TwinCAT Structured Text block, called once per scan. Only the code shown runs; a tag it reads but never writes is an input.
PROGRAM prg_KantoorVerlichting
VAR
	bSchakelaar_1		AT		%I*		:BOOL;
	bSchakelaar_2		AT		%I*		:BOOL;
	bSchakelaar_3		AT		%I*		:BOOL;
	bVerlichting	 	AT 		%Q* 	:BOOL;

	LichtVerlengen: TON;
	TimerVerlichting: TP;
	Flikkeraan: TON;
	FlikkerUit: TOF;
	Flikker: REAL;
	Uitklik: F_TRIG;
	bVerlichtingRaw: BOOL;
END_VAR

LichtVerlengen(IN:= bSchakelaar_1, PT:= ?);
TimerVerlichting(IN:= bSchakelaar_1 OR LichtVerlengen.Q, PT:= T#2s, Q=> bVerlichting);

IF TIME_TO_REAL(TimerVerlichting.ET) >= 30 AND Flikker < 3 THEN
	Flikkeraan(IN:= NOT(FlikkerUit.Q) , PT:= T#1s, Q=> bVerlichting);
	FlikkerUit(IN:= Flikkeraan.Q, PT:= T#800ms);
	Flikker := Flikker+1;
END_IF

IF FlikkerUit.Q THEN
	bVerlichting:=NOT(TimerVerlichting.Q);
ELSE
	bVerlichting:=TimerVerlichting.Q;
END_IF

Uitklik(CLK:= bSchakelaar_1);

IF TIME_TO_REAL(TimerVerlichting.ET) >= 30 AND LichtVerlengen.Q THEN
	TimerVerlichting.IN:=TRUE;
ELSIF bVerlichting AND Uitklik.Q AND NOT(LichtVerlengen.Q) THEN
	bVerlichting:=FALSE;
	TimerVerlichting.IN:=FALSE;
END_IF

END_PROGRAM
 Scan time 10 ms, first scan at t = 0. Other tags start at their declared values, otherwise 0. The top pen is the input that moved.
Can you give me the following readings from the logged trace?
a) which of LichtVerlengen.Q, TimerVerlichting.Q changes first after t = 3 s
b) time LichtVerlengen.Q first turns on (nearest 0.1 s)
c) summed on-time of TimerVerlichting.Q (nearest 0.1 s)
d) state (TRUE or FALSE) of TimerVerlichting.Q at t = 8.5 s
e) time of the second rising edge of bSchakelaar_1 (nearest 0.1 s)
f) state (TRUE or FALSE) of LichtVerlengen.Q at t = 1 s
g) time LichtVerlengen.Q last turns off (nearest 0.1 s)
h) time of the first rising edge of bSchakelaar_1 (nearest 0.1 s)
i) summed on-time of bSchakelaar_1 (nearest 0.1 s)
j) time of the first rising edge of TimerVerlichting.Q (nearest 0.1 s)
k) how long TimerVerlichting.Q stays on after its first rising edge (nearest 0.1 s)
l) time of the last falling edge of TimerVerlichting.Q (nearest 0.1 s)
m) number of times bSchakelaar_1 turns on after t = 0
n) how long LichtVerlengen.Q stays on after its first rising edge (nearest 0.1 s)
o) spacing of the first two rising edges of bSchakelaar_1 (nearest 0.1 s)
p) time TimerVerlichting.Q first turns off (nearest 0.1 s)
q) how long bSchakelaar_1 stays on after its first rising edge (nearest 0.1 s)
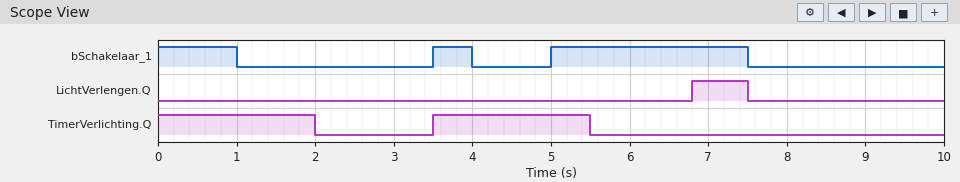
TimerVerlichting.Q
6.8 s
4.0 s
FALSE
5.0 s
FALSE
7.5 s
3.5 s
4.0 s
3.5 s
2.0 s
5.5 s
2
0.7 s
1.5 s
2.0 s
0.5 s
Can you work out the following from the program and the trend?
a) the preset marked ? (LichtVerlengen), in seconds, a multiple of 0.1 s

1.8 s
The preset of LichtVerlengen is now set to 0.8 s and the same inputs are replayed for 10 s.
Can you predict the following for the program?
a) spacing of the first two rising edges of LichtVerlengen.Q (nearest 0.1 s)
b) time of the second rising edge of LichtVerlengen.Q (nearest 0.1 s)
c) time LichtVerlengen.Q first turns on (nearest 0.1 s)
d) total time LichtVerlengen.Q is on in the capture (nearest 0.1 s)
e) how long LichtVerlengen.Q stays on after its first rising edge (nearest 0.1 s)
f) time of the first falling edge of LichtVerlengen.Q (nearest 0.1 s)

5.0 s
5.8 s
0.8 s
1.9 s
0.2 s
1.0 s
